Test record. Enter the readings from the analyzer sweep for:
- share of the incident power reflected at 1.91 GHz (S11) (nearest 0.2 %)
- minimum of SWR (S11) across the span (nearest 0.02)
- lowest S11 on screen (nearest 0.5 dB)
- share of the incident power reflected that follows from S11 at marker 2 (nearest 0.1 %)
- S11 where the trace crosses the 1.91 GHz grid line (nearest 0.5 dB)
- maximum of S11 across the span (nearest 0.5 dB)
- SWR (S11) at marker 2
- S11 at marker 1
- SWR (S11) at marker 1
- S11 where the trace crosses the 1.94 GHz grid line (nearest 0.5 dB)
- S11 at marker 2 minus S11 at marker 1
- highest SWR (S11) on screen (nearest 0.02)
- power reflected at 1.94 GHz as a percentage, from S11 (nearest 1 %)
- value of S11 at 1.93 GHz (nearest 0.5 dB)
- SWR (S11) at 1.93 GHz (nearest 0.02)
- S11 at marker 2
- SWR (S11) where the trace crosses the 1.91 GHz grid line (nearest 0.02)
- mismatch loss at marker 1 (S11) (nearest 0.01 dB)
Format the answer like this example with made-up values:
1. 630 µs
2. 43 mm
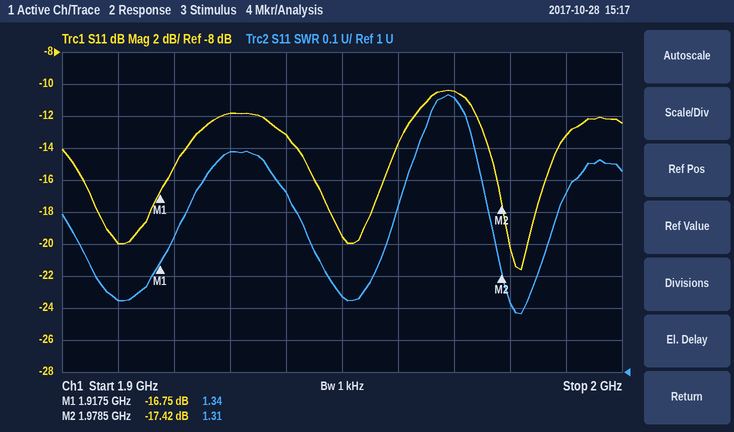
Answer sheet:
1. 1.0 %
2. 1.18
3. -21.5 dB
4. 1.8 %
5. -20.0 dB
6. -10.5 dB
7. 1.31
8. -16.75 dB
9. 1.34
10. -13.0 dB
11. -0.67 dB
12. 1.86
13. 5 %
14. -12.0 dB
15. 1.68
16. -17.42 dB
17. 1.22
18. 0.09 dB
